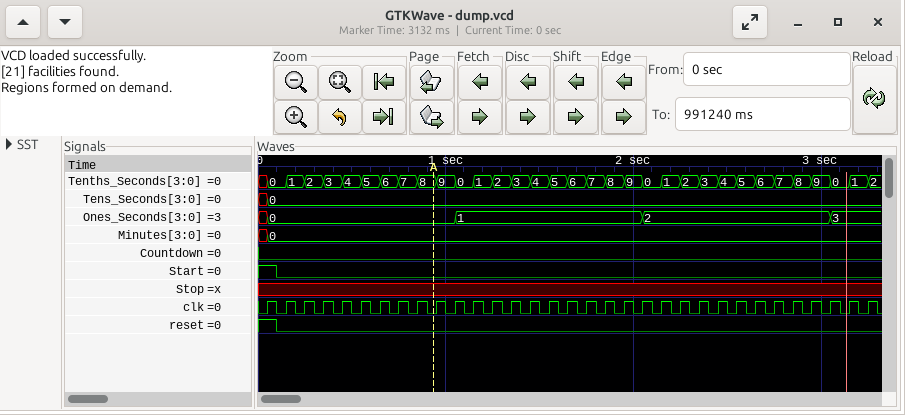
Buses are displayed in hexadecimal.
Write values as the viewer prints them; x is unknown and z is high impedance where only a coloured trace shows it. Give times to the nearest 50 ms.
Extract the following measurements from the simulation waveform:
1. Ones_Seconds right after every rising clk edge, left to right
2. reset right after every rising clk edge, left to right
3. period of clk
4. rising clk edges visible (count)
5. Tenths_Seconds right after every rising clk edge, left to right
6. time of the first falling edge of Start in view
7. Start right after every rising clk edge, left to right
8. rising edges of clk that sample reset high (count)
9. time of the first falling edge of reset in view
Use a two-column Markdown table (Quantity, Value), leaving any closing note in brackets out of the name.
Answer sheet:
| Quantity | Value |
|---|---|
| Ones_Seconds right after every rising clk edge, left to right | 0, 0, 0, 0, 0, 0, 0, 0, 0, 0, 1, 1, 1, 1, 1, 1, 1, 1, 1, 1, 2, 2, 2, 2, 2, 2, 2, 2, 2, 2, 3, 3, 3 |
| reset right after every rising clk edge, left to right | 1 0 0 0 0 0 0 0 0 0 0 0 0 0 0 0 0 0 0 0 0 0 0 0 0 0 0 0 0 0 0 0 0 |
| period of clk | 100 ms |
| rising clk edges visible | 33 |
| Tenths_Seconds right after every rising clk edge, left to right | 0, 1, 2, 3, 4, 5, 6, 7, 8, 9, 0, 1, 2, 3, 4, 5, 6, 7, 8, 9, 0, 1, 2, 3, 4, 5, 6, 7, 8, 9, 0, 1, 2 |
| time of the first falling edge of Start in view | 100 ms |
| Start right after every rising clk edge, left to right | 1 0 0 0 0 0 0 0 0 0 0 0 0 0 0 0 0 0 0 0 0 0 0 0 0 0 0 0 0 0 0 0 0 |
| rising edges of clk that sample reset high | 1 |
| time of the first falling edge of reset in view | 100 ms |
